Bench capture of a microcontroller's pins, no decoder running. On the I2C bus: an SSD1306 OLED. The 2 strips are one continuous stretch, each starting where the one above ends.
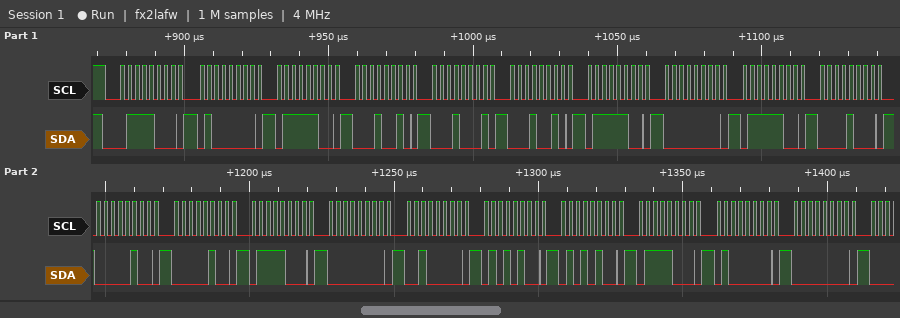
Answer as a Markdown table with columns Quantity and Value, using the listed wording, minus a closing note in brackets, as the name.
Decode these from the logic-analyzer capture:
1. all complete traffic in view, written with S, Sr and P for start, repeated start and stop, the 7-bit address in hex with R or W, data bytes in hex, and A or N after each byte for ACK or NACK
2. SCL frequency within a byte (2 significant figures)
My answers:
| Quantity | Value |
|---|---|
| all complete traffic in view, written with S, Sr and P for start, repeated start and stop, the 7-bit address in hex with R or W, data bytes in hex, and A or N after each byte for ACK or NACK | S 3CW A 40 A 7C A 12 A 11 A 12 A 7C A 00 A 7C A 08 A 04 A 04 A 78 A 00 A 20 A 54 A 54 A 78 A 40 A 00 A |
| SCL frequency within a byte | 400 kHz |
